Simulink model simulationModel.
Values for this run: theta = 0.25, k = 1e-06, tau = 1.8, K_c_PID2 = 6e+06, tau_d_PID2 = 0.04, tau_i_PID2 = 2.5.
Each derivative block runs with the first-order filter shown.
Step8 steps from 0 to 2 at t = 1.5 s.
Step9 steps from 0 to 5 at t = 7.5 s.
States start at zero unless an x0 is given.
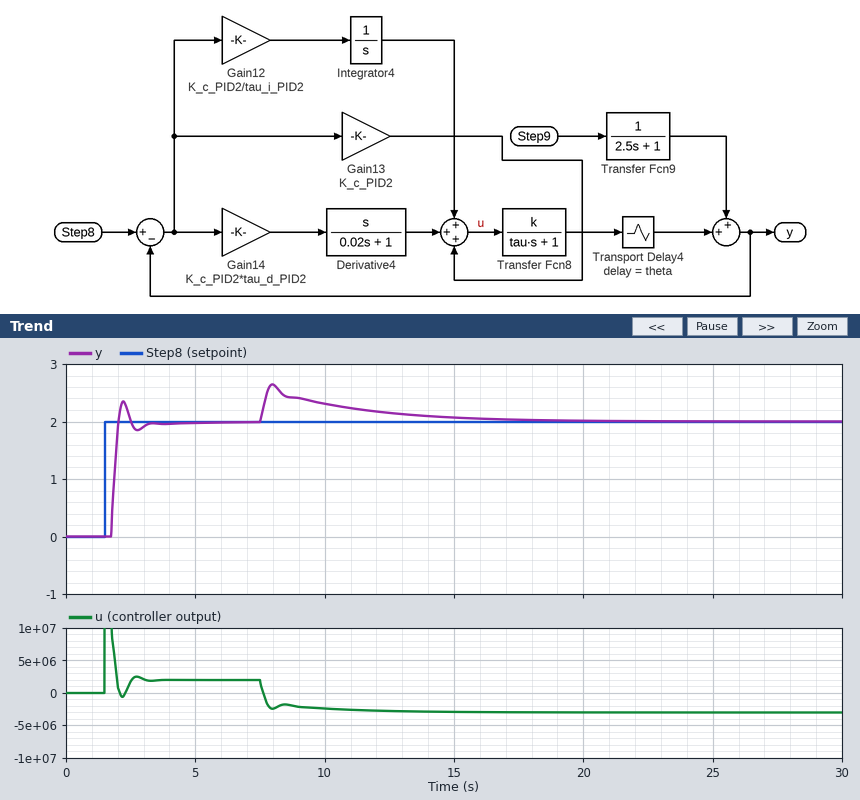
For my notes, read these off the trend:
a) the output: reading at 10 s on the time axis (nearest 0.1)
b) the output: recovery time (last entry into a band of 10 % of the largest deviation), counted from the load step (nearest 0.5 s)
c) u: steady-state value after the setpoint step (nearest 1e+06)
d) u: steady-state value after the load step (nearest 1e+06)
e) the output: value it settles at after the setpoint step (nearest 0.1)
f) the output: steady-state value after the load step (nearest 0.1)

2.3
7.5 s
2000000
-3000000
2.0
2.0
